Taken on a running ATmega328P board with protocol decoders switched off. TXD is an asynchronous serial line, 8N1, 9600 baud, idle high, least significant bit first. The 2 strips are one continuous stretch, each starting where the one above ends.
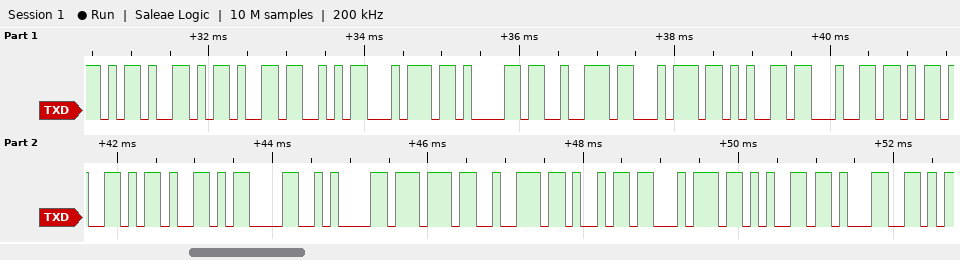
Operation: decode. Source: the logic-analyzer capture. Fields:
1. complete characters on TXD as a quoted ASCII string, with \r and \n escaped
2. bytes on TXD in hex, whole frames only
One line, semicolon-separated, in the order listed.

"--Started--\r\nwrite1"; 2D 2D 53 74 61 72 74 65 64 2D 2D 0D 0A 77 72 69 74 65 31
